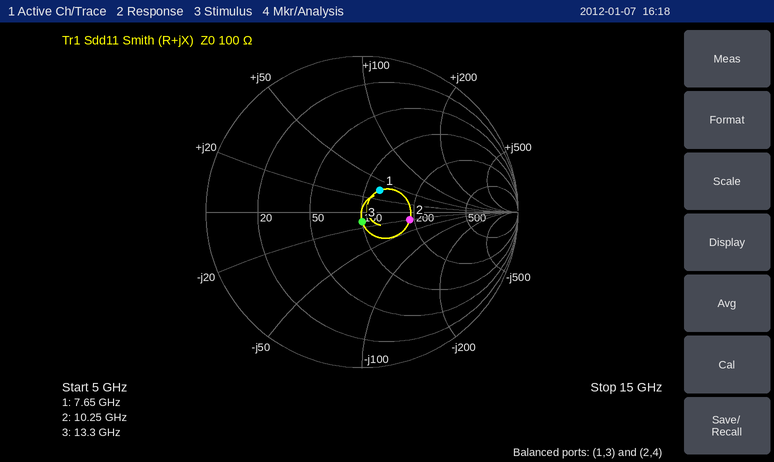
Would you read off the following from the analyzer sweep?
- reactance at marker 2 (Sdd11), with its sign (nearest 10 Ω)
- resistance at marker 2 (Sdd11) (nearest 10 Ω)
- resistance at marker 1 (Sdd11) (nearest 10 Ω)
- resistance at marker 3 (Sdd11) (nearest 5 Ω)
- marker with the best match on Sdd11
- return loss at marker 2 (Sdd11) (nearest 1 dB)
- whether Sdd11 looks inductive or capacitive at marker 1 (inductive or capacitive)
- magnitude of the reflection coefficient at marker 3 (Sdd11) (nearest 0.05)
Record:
-20 Ω
190 Ω
120 Ω
100 Ω
marker 3
10 dB
inductive
0.05
